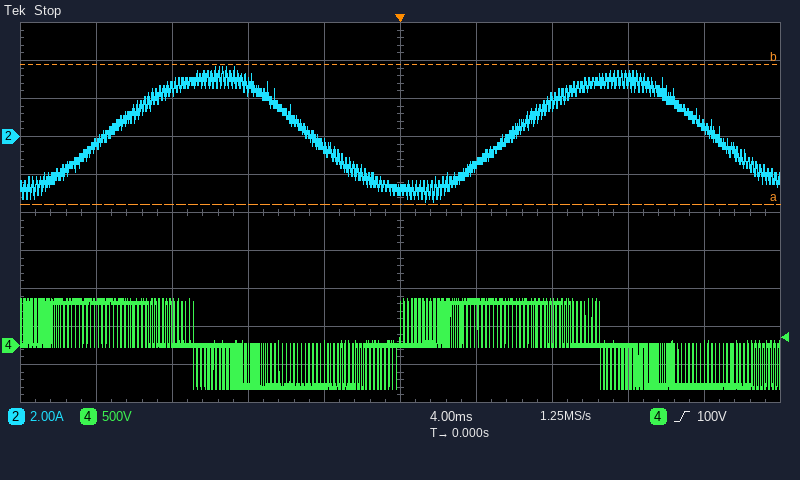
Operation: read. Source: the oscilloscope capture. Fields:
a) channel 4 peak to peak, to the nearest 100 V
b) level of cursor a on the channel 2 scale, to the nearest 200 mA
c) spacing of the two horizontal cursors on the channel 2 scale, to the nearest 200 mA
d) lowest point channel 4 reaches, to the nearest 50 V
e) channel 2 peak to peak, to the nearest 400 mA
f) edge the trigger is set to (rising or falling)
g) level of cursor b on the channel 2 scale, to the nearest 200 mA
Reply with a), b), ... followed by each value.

a) 1.20 kV
b) -3.6 A
c) 7.4 A
d) -600 V
e) 7.2 A
f) rising
g) 3.8 A
